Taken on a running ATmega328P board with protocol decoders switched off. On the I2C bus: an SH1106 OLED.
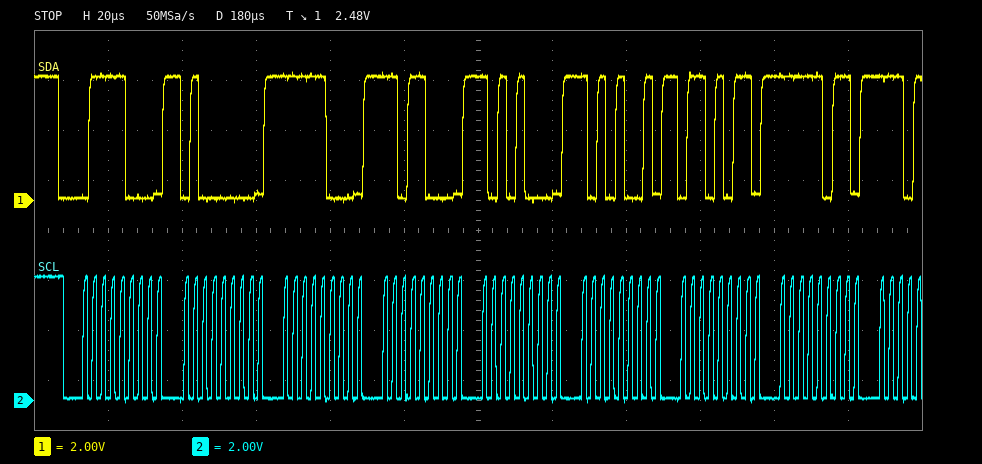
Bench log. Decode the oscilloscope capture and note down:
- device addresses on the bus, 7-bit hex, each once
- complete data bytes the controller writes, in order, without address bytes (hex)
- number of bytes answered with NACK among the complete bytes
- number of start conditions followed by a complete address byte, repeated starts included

0x3C
40 F8 D8 A8 A9 6B FB
0
1
